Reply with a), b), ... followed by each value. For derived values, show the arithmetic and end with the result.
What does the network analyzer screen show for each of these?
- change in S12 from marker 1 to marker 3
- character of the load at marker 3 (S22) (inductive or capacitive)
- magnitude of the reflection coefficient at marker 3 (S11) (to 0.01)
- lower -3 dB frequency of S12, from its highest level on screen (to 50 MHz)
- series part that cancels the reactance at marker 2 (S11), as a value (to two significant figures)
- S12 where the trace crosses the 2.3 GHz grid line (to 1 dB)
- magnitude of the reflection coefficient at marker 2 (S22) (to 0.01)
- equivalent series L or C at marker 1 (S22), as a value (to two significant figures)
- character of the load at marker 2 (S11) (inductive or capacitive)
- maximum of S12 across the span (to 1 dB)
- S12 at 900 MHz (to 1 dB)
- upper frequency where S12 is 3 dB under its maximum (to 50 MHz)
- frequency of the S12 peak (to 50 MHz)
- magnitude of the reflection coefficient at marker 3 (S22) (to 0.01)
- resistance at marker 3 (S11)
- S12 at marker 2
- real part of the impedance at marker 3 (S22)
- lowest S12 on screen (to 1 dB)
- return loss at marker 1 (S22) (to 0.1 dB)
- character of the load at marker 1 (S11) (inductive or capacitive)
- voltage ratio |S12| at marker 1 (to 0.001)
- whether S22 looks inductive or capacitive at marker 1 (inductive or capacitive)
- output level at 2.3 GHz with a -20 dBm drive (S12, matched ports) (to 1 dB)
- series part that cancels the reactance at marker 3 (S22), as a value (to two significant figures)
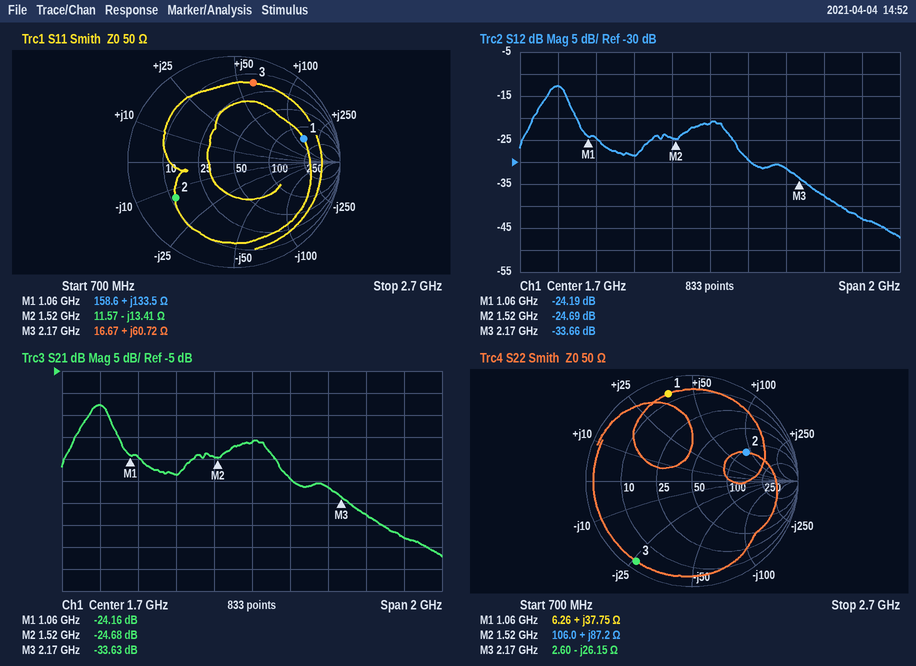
a) -33.66 − (-24.19) = -9.47 dB
b) capacitive
c) 0.77
d) 850 MHz
e) L = 13.41 Ω/(2π × 1.52 GHz) ≈ 1.4 nH
f) -38 dB
g) 0.58
h) L = 37.75 Ω/(2π × 1.06 GHz) ≈ 5.7 nH
i) capacitive
j) -13 dB
k) -13 dB
l) 950 MHz
m) 900 MHz
n) 0.92
o) 16.67 Ω
p) -24.69 dB
q) 2.60 Ω
r) -47 dB
s) 1.4 dB
t) inductive
u) 10^(-24.19/20) ≈ 0.062
v) inductive
w) -20 dBm + (-38 dB) = -58 dBm
x) L = 26.15 Ω/(2π × 2.17 GHz) ≈ 1.9 nH
